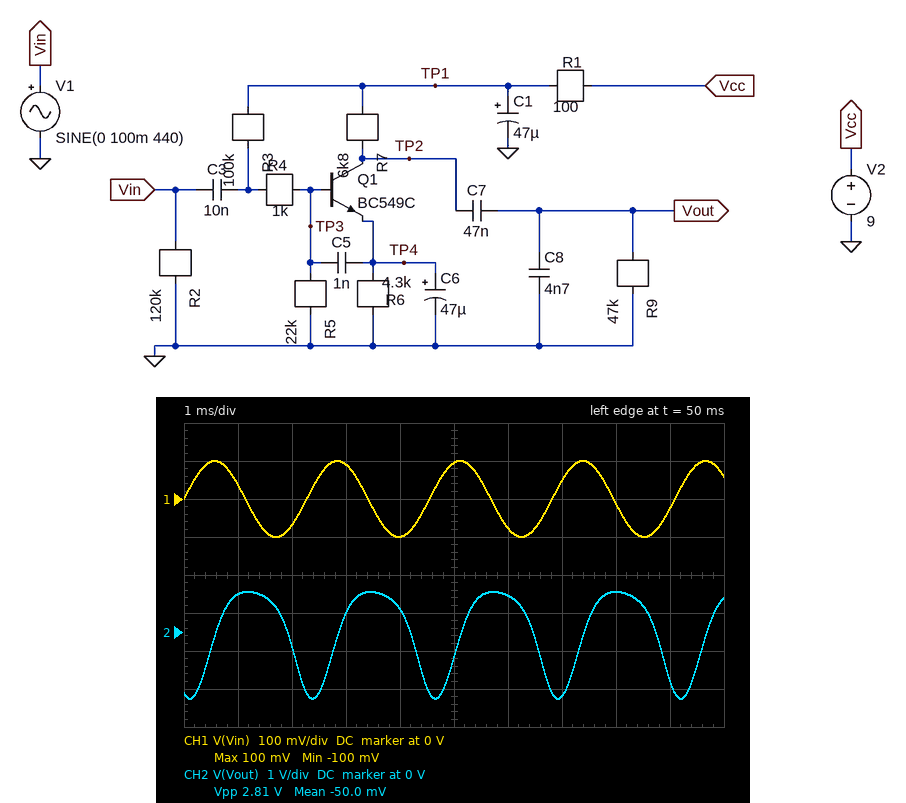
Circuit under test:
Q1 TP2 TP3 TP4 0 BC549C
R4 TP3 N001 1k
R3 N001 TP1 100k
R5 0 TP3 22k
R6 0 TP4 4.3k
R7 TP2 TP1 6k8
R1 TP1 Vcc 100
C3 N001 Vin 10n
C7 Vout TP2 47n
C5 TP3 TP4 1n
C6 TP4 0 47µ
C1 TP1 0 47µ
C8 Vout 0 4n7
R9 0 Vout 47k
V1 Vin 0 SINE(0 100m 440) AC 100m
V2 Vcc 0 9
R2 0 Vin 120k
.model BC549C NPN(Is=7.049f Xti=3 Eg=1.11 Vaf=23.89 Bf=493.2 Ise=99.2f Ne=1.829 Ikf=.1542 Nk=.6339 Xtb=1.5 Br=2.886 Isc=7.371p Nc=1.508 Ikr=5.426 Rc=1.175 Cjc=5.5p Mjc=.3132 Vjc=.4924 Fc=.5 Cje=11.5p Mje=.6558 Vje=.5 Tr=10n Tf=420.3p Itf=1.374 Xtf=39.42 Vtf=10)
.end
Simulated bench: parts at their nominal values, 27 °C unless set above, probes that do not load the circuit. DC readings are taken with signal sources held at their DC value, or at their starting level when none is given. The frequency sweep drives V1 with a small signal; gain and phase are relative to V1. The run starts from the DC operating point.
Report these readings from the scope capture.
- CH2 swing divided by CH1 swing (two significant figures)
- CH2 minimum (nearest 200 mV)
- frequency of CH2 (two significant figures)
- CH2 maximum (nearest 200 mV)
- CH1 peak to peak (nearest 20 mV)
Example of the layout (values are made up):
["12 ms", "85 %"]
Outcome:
["14", "-1.8 V", "440 Hz", "1.0 V", "200 mV"]
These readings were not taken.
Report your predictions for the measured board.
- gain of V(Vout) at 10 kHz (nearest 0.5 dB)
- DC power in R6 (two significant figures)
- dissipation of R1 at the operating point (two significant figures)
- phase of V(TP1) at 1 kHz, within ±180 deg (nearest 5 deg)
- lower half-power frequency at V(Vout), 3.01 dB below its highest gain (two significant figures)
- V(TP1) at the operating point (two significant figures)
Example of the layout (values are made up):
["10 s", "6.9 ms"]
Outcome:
["26.5 dB", "220 µW", "9.0 µW", "130 deg", "770 Hz", "9.0 V"]
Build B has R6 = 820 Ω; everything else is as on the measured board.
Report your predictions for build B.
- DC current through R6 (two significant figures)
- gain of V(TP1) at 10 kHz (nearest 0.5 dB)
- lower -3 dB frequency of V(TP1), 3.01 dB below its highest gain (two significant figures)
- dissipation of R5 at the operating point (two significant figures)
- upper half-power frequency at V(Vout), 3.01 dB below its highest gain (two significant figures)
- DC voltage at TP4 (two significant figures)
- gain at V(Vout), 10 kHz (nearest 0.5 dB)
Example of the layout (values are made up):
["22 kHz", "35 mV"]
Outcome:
["1.1 mA", "-47.0 dB", "61 Hz", "110 µW", "11 kHz", "880 mV", "38.5 dB"]
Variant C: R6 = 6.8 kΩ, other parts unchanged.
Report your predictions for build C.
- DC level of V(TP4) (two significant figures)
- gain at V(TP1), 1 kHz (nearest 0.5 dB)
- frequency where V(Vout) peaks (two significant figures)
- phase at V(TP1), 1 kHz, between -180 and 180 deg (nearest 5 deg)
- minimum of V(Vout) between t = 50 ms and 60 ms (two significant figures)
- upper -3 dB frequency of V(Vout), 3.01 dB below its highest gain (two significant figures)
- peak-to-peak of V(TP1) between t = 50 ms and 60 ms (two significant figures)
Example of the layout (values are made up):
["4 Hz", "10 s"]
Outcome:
["990 mV", "-39.5 dB", "2.4 kHz", "125 deg", "-1.3 V", "8.0 kHz", "2.4 mV"]
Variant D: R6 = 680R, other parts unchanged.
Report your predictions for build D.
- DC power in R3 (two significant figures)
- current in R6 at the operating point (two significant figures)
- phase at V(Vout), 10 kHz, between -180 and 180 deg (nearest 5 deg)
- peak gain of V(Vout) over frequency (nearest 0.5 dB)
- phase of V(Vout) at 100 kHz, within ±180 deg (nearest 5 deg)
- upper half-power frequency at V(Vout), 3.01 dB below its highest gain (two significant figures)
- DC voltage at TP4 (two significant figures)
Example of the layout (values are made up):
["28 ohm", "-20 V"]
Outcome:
["540 µW", "1.2 mA", "-125 deg", "17.5 dB", "140 deg", "190 kHz", "800 mV"]
